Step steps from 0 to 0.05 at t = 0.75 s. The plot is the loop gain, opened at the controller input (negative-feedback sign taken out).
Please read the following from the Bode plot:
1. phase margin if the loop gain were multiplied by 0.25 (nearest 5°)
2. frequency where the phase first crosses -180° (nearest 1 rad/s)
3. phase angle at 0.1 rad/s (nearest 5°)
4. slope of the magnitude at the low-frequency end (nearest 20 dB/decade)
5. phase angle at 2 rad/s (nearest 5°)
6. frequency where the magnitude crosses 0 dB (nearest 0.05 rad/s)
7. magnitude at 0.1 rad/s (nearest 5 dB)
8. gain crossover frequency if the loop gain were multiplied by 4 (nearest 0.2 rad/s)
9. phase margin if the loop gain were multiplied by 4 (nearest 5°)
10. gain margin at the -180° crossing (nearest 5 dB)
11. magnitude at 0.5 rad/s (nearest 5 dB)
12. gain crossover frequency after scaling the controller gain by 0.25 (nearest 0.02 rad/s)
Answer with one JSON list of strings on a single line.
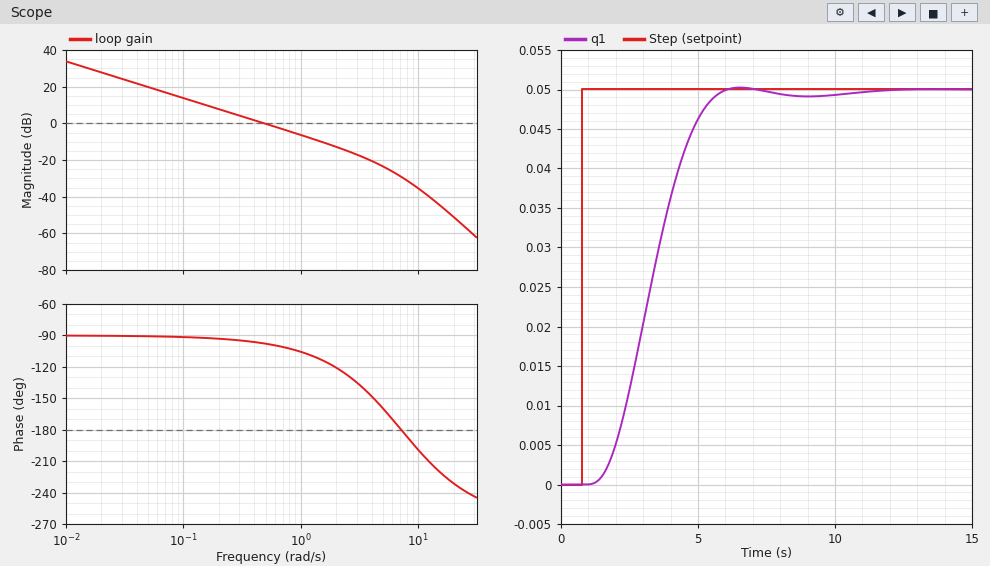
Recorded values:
["90°", "7 rad/s", "-90°", "-20 dB/decade", "-120°", "0.50 rad/s", "15 dB", "1.8 rad/s", "60°", "30 dB", "0 dB", "0.12 rad/s"]
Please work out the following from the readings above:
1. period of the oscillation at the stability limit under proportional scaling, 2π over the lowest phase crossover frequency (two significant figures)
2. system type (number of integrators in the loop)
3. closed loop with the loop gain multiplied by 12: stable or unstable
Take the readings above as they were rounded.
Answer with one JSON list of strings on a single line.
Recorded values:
["0.90 s", "1", "stable"]
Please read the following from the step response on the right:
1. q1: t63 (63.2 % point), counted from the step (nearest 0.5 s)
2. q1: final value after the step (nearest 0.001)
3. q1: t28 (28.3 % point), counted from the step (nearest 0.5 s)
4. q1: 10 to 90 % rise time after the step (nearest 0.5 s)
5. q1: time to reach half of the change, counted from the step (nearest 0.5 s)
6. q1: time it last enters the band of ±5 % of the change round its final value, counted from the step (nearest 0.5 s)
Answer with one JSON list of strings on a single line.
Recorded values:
["3.0 s", "0.050", "2.0 s", "3.0 s", "2.5 s", "4.5 s"]
